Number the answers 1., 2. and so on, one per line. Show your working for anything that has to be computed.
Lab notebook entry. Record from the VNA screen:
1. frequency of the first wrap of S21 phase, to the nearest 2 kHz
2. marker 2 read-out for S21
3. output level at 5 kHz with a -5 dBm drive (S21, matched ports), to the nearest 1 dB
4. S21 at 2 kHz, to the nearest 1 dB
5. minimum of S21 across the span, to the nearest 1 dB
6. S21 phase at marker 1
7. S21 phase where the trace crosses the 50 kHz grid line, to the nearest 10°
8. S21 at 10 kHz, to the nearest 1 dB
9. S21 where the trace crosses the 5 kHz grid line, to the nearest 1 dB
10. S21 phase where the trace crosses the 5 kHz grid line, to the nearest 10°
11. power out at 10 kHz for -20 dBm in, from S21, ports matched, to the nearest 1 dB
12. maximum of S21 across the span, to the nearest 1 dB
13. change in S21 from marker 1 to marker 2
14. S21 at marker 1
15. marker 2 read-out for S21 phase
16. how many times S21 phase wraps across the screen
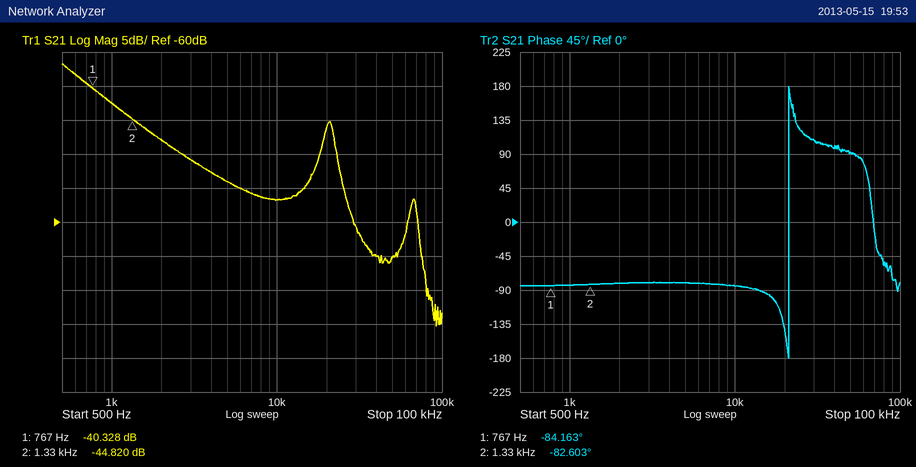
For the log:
1. 22 kHz
2. -44.820 dB
3. -5 dBm + (-54 dB) = -59 dBm
4. -48 dB
5. -75 dB
6. -84.163°
7. 90°
8. -57 dB
9. -54 dB
10. -80°
11. -20 dBm + (-57 dB) = -77 dBm
12. -37 dB
13. -44.82 − (-40.328) = -4.492 dB
14. -40.328 dB
15. -82.603°
16. 1
